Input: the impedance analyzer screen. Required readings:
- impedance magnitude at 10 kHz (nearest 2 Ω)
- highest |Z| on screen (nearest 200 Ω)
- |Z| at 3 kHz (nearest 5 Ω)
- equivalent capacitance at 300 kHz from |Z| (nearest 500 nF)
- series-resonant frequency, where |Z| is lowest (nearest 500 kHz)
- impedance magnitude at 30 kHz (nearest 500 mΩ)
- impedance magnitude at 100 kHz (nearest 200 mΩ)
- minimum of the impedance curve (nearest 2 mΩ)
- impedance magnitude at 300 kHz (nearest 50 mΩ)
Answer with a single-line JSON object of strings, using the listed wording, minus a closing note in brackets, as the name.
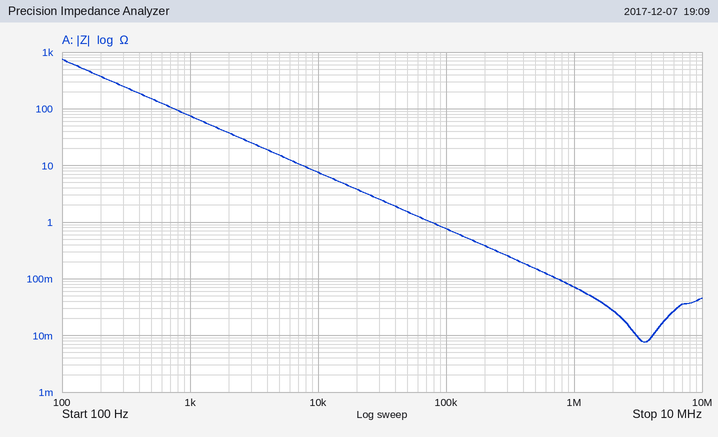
{"impedance magnitude at 10 kHz": "8 Ω", "highest |Z| on screen": "800 Ω", "|Z| at 3 kHz": "25 Ω", "equivalent capacitance at 300 kHz from |Z|": "2.0 µF", "series-resonant frequency, where |Z| is lowest": "3.5 MHz", "impedance magnitude at 30 kHz": "2.5 Ω", "impedance magnitude at 100 kHz": "800 mΩ", "minimum of the impedance curve": "8 mΩ", "impedance magnitude at 300 kHz": "250 mΩ"}
